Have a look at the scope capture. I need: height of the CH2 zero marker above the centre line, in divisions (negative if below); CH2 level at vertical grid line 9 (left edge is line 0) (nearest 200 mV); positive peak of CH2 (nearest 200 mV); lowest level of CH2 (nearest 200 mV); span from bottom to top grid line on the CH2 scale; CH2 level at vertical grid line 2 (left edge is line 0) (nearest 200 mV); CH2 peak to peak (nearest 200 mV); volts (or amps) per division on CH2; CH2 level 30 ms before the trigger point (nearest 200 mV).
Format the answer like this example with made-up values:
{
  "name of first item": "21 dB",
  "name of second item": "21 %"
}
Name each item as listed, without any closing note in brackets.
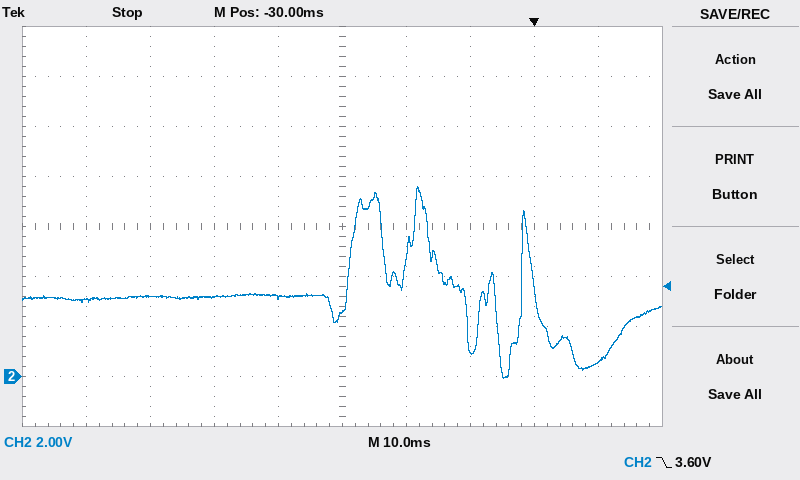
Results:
{
  "height of the CH2 zero marker above the centre line, in divisions": "-3.0 div",
  "CH2 level at vertical grid line 9 (left edge is line 0)": "600 mV",
  "positive peak of CH2": "7.6 V",
  "lowest level of CH2": "0.0 V",
  "span from bottom to top grid line on the CH2 scale": "16 V",
  "CH2 level at vertical grid line 2 (left edge is line 0)": "3.2 V",
  "CH2 peak to peak": "7.6 V",
  "volts (or amps) per division on CH2": "2 V",
  "CH2 level 30 ms before the trigger point": "2.6 V"
}
